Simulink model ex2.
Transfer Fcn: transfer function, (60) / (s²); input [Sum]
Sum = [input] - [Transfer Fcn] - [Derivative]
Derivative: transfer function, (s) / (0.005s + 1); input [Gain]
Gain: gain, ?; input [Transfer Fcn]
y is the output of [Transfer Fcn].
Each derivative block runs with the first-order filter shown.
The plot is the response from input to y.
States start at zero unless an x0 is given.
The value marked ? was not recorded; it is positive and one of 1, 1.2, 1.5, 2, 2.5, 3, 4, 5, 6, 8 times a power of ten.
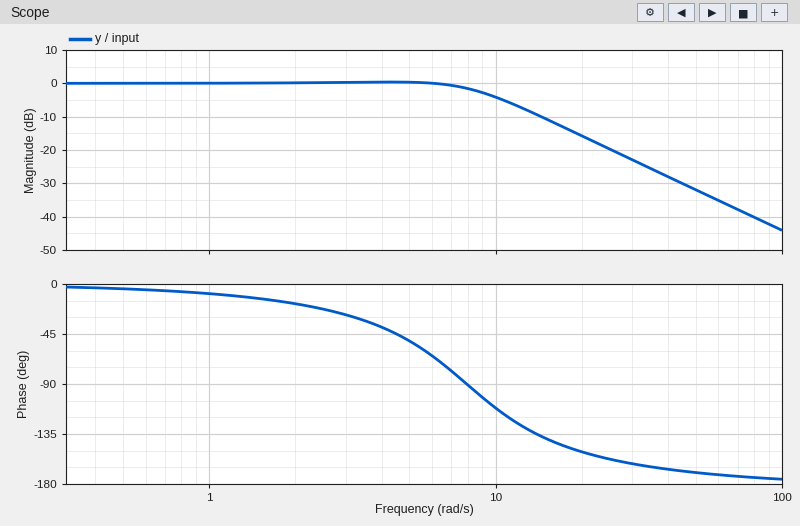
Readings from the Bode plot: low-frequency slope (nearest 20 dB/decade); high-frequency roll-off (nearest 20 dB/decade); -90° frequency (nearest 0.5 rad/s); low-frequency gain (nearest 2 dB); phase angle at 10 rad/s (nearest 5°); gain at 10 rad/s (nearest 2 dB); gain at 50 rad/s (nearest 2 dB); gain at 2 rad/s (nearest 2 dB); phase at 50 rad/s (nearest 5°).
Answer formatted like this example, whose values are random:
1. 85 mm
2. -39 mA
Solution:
1. 0 dB/decade
2. -40 dB/decade
3. 8.0 rad/s
4. 0 dB
5. -110°
6. -4 dB
7. -32 dB
8. 0 dB
9. -170°
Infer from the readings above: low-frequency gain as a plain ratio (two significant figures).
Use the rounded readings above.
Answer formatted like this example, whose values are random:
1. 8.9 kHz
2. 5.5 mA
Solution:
1. 1.0
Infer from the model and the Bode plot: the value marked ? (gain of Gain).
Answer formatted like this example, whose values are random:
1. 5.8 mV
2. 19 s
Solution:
1. 0.15
